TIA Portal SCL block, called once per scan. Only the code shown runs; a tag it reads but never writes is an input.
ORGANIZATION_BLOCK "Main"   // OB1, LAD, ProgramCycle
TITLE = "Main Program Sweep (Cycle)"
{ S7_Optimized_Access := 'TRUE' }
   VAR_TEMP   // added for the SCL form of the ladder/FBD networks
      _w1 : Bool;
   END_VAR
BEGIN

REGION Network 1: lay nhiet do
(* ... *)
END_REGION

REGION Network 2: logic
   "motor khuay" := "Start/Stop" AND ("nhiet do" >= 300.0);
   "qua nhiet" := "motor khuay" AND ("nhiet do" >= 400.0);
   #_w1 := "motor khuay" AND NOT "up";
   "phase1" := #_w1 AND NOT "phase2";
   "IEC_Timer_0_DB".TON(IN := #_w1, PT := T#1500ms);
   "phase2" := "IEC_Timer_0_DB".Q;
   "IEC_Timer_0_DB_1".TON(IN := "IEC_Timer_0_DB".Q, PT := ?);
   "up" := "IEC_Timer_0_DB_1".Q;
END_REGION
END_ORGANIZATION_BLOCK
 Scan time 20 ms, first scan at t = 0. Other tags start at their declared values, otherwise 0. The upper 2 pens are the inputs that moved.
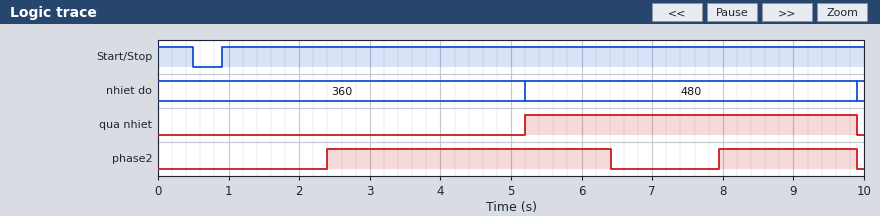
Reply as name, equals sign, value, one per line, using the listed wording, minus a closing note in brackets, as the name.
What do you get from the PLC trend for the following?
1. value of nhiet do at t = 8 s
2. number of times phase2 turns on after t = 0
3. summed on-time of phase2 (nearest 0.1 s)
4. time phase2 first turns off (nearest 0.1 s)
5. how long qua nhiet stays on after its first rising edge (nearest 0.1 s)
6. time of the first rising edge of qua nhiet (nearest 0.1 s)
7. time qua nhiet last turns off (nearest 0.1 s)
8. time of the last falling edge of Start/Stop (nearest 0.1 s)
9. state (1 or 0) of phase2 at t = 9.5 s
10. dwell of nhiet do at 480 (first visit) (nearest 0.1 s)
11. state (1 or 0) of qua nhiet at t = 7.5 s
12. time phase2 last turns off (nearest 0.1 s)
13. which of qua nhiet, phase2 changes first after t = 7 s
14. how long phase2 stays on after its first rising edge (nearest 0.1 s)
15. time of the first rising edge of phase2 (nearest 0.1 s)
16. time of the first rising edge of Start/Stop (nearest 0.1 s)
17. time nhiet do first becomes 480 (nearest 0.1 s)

value of nhiet do at t = 8 s = 480
number of times phase2 turns on after t = 0 = 2
summed on-time of phase2 = 6.0 s
time phase2 first turns off = 6.4 s
how long qua nhiet stays on after its first rising edge = 4.7 s
time of the first rising edge of qua nhiet = 5.2 s
time qua nhiet last turns off = 9.9 s
time of the last falling edge of Start/Stop = 0.5 s
state (1 or 0) of phase2 at t = 9.5 s = 1
dwell of nhiet do at 480 (first visit) = 4.7 s
state (1 or 0) of qua nhiet at t = 7.5 s = 1
time phase2 last turns off = 9.9 s
which of qua nhiet, phase2 changes first after t = 7 s = phase2
how long phase2 stays on after its first rising edge = 4.0 s
time of the first rising edge of phase2 = 2.4 s
time of the first rising edge of Start/Stop = 0.9 s
time nhiet do first becomes 480 = 5.2 s
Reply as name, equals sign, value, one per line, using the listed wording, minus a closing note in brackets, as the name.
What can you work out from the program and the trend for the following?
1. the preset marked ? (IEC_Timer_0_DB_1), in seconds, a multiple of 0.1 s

the preset marked ? (IEC_Timer_0_DB_1), in seconds, a multiple of 0.1 s = 4.0 s
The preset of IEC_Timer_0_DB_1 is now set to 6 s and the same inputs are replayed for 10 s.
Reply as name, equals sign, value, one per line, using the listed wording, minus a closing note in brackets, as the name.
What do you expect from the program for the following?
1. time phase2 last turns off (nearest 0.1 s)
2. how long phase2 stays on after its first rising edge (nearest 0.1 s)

time phase2 last turns off = 8.4 s
how long phase2 stays on after its first rising edge = 6.0 s
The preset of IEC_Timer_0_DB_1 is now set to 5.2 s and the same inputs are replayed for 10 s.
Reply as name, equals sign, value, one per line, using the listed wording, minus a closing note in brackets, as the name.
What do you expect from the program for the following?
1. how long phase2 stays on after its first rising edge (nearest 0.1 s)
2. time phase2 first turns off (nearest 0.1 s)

how long phase2 stays on after its first rising edge = 5.2 s
time phase2 first turns off = 7.6 s
